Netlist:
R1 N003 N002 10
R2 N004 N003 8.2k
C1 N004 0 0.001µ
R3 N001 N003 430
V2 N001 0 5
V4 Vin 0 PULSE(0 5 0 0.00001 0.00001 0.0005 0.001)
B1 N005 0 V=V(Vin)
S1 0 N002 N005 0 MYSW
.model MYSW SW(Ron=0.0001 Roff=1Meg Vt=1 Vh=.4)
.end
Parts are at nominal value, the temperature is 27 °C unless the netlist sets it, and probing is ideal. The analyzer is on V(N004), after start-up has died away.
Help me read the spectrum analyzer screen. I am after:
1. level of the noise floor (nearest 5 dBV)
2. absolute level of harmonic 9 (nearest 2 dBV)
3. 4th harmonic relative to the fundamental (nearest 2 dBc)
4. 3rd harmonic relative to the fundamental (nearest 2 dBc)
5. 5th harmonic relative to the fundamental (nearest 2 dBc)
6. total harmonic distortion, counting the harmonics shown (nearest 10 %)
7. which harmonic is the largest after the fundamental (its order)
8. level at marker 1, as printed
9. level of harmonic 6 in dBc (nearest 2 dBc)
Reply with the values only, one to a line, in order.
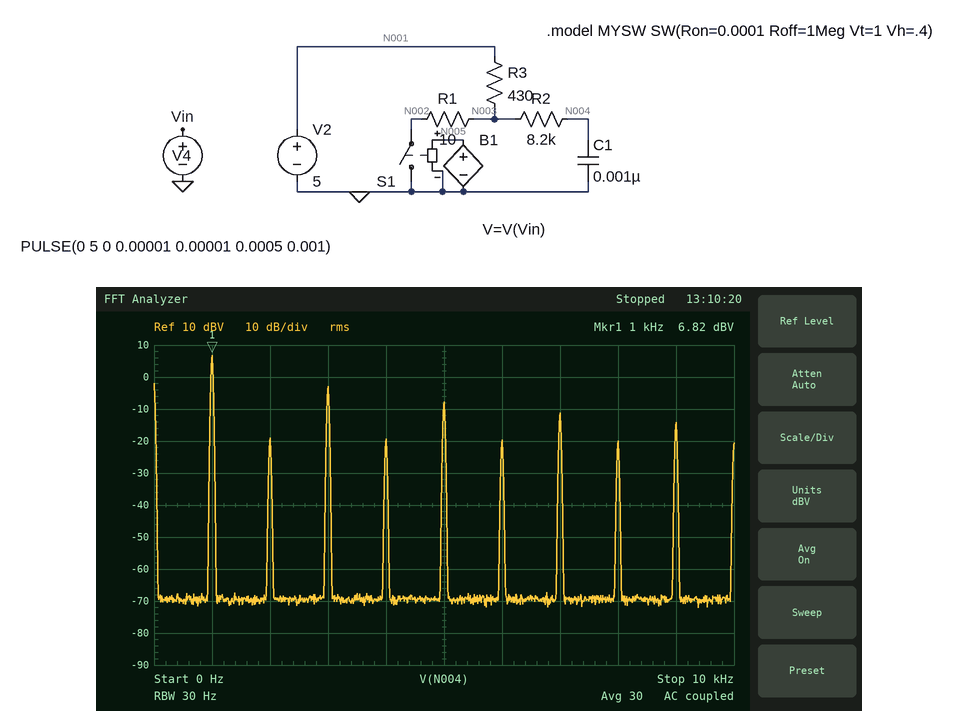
-70 dBV
-14 dBV
-26 dBc
-10 dBc
-14 dBc
40 %
3
6.82 dBV
-26 dBc
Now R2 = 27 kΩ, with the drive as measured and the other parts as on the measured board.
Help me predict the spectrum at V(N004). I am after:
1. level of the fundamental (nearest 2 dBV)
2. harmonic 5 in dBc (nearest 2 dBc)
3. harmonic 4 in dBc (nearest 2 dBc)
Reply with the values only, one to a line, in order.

6 dBV
-16 dBc
-28 dBc
